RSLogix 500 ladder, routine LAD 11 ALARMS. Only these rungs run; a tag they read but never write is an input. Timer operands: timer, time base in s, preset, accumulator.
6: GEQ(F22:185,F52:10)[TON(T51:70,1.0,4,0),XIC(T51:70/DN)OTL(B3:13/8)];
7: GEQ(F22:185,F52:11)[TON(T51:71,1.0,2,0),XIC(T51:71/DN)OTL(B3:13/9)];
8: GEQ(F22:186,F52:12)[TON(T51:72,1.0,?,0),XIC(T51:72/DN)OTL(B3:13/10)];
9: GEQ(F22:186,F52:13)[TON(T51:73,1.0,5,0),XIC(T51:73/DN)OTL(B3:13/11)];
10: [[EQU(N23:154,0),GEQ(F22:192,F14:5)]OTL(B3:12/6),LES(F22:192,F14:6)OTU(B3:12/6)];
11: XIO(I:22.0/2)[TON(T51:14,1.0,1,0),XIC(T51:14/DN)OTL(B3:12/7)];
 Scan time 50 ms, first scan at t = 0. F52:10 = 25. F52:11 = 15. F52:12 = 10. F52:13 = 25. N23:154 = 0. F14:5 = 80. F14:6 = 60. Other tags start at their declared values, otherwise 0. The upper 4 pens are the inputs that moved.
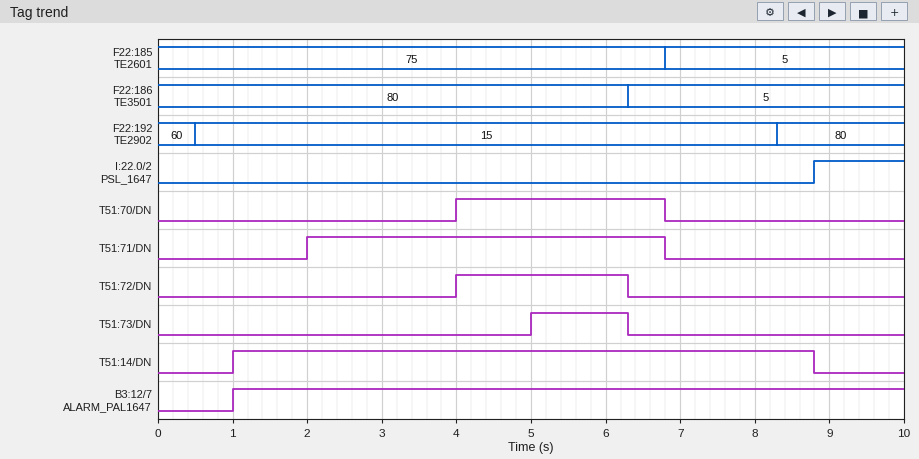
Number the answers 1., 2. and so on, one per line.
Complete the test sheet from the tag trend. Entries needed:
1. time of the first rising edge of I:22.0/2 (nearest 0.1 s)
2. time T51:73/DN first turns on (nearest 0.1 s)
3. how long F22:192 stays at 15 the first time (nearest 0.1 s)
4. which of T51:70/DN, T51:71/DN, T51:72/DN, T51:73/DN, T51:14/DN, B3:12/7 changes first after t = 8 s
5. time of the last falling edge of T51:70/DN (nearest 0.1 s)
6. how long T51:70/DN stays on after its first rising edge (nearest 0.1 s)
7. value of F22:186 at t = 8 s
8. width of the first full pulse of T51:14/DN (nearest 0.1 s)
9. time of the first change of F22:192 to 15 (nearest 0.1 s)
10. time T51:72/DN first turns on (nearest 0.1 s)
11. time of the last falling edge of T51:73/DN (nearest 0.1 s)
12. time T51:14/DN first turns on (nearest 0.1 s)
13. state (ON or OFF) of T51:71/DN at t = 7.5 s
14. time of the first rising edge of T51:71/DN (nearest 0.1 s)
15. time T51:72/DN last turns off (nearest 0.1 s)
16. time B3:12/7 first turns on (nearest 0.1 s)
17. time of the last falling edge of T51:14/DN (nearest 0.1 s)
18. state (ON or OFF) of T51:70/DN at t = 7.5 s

1. 8.8 s
2. 5.0 s
3. 7.8 s
4. T51:14/DN
5. 6.8 s
6. 2.8 s
7. 5
8. 7.8 s
9. 0.5 s
10. 4.0 s
11. 6.3 s
12. 1.0 s
13. OFF
14. 2.0 s
15. 6.3 s
16. 1.0 s
17. 8.8 s
18. OFF
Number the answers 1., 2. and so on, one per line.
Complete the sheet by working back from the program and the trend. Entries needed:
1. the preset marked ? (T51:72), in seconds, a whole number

1. 4 s
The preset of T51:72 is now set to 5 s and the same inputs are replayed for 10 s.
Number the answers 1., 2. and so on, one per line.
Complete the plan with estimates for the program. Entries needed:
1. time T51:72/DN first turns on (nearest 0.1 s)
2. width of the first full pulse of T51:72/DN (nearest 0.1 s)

1. 5.0 s
2. 1.3 s
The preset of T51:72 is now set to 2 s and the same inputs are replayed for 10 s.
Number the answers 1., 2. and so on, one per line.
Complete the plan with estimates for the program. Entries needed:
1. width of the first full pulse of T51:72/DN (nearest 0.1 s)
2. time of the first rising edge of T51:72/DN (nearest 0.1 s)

1. 4.3 s
2. 2.0 s
